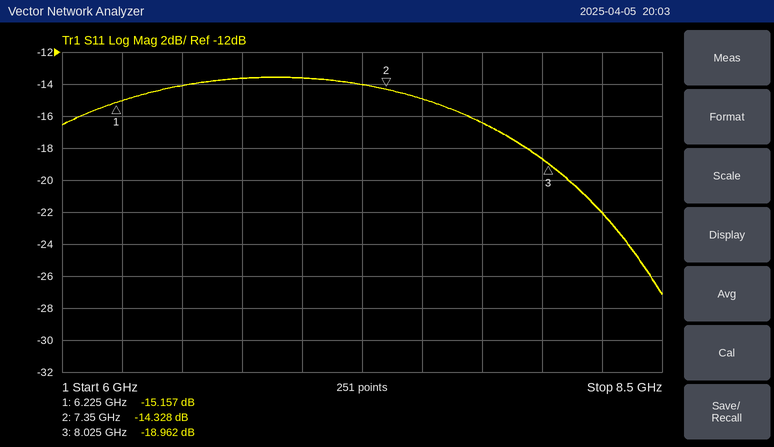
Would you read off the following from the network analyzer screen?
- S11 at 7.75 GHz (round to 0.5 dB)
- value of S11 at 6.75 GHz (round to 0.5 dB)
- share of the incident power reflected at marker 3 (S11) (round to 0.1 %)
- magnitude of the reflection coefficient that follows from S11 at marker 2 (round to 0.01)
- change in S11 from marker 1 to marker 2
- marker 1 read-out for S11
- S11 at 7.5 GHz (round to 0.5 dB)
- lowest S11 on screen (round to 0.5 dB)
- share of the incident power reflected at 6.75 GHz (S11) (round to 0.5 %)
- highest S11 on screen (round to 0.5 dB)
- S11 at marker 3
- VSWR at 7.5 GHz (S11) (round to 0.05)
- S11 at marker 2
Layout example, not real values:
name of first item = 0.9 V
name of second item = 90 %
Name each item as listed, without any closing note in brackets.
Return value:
S11 at 7.75 GHz = -16.5 dB
value of S11 at 6.75 GHz = -13.5 dB
share of the incident power reflected at marker 3 (S11) = 1.3 %
magnitude of the reflection coefficient that follows from S11 at marker 2 = 0.19
change in S11 from marker 1 to marker 2 = 0.829 dB
marker 1 read-out for S11 = -15.157 dB
S11 at 7.5 GHz = -15.0 dB
lowest S11 on screen = -27.0 dB
share of the incident power reflected at 6.75 GHz (S11) = 4.5 %
highest S11 on screen = -13.5 dB
S11 at marker 3 = -18.962 dB
VSWR at 7.5 GHz (S11) = 1.45
S11 at marker 2 = -14.328 dB
